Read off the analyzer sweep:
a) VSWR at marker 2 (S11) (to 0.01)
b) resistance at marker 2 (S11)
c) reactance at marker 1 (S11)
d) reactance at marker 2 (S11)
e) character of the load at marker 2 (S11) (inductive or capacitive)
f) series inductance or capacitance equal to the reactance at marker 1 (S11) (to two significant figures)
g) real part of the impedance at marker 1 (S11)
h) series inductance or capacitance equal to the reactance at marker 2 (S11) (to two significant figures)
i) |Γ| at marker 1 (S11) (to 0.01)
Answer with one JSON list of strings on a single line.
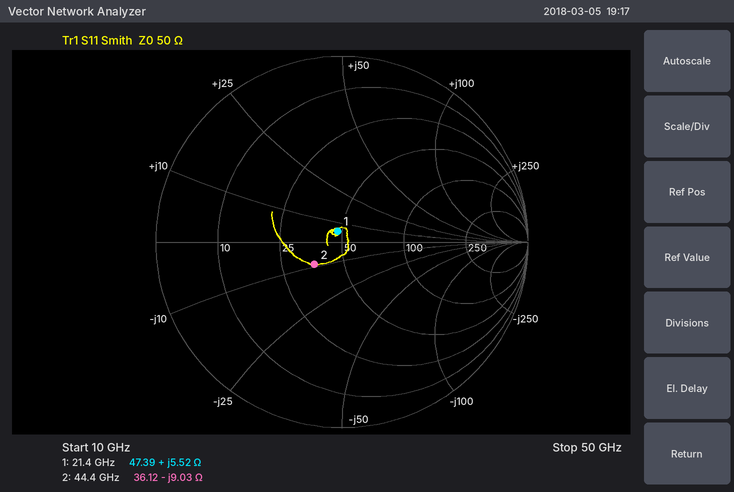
["1.47", "36.12 Ω", "+5.52 Ω", "-9.03 Ω", "capacitive", "41 pH", "47.39 Ω", "400 fF", "0.06"]
